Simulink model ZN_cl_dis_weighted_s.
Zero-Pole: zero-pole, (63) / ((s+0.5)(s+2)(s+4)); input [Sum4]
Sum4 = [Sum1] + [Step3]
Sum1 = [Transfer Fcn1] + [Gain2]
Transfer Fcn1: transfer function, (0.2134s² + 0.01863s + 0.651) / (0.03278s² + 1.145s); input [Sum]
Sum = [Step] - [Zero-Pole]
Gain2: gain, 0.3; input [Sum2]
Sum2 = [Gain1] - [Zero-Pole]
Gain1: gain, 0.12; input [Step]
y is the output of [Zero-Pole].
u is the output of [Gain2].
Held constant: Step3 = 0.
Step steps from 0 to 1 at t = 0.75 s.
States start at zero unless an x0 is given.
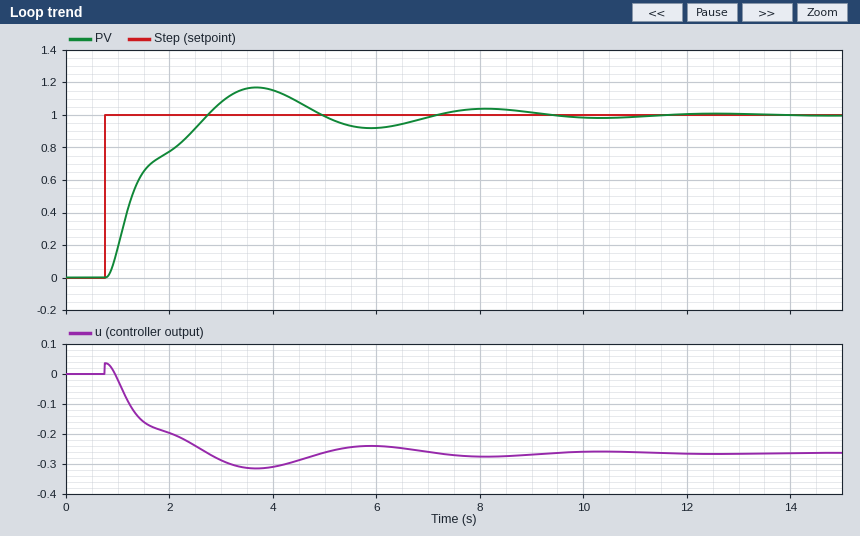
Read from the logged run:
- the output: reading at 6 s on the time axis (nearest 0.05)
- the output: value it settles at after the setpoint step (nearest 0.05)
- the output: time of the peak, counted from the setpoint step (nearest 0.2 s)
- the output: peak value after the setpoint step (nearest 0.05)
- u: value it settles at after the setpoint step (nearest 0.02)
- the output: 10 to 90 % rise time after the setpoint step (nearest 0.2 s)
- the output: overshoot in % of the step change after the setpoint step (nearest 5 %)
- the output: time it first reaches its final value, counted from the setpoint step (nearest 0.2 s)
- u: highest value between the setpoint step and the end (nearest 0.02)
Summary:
0.90
1.00
3.0 s
1.15
-0.26
1.6 s
15 %
2.0 s
0.04
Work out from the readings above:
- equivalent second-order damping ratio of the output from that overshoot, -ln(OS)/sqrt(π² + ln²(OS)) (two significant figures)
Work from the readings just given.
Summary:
0.52
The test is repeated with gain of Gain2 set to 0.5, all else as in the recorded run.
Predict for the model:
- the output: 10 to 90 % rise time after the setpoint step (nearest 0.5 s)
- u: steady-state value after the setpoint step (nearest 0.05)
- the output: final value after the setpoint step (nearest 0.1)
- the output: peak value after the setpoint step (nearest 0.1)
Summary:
2.0 s
-0.45
1.0
1.1
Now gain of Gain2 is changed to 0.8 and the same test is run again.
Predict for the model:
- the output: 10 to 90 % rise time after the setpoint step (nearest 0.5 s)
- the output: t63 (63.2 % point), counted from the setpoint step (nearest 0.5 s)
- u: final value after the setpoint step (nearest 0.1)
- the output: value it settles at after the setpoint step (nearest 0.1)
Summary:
2.5 s
2.0 s
-0.7
1.0
